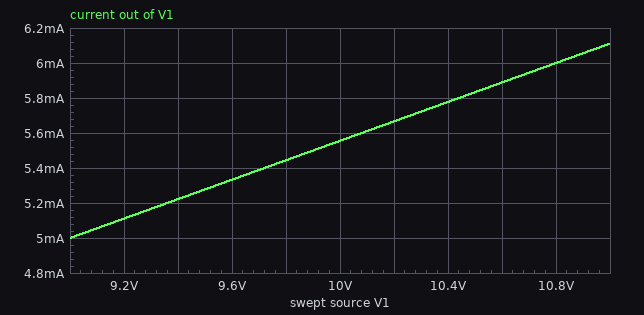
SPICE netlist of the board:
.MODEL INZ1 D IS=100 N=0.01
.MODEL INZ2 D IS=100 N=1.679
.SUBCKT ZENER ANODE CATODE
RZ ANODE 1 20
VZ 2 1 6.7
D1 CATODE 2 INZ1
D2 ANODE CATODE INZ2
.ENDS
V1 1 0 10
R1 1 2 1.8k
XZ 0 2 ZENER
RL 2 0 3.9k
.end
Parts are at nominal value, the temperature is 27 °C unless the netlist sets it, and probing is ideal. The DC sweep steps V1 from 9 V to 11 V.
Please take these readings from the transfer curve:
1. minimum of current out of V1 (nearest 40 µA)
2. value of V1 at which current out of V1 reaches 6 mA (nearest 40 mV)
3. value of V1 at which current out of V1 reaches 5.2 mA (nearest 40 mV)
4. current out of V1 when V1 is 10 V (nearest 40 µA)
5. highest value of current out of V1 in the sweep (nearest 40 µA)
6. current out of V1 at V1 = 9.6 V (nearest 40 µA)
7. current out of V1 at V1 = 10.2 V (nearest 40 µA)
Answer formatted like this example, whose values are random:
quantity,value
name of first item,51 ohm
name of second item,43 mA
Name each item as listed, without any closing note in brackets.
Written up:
quantity,value
minimum of current out of V1,5.00 mA
value of V1 at which current out of V1 reaches 6 mA,10.80 V
value of V1 at which current out of V1 reaches 5.2 mA,9.36 V
current out of V1 when V1 is 10 V,5.56 mA
highest value of current out of V1 in the sweep,6.12 mA
current out of V1 at V1 = 9.6 V,5.32 mA
current out of V1 at V1 = 10.2 V,5.68 mA
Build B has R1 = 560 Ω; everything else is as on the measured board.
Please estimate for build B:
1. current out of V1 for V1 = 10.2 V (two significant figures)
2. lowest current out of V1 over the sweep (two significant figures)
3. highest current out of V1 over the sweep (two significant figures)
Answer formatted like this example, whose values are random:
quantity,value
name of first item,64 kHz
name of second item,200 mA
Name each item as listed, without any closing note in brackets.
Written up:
quantity,value
current out of V1 for V1 = 10.2 V,18 mA
lowest current out of V1 over the sweep,16 mA
highest current out of V1 over the sweep,20 mA
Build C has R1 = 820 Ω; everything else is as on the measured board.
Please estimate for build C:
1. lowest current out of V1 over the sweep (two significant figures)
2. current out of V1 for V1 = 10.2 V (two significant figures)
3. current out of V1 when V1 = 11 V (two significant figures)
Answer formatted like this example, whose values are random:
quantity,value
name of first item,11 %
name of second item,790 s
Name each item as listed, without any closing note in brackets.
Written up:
quantity,value
lowest current out of V1 over the sweep,11 mA
current out of V1 for V1 = 10.2 V,12 mA
current out of V1 when V1 = 11 V,13 mA
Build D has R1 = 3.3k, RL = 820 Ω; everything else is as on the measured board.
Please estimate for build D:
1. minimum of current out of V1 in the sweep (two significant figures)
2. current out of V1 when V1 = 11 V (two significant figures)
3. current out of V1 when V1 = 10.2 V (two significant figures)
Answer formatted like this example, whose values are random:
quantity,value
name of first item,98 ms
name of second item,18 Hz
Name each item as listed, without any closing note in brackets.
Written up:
quantity,value
minimum of current out of V1 in the sweep,2.7 mA
current out of V1 when V1 = 11 V,3.3 mA
current out of V1 when V1 = 10.2 V,3.1 mA
